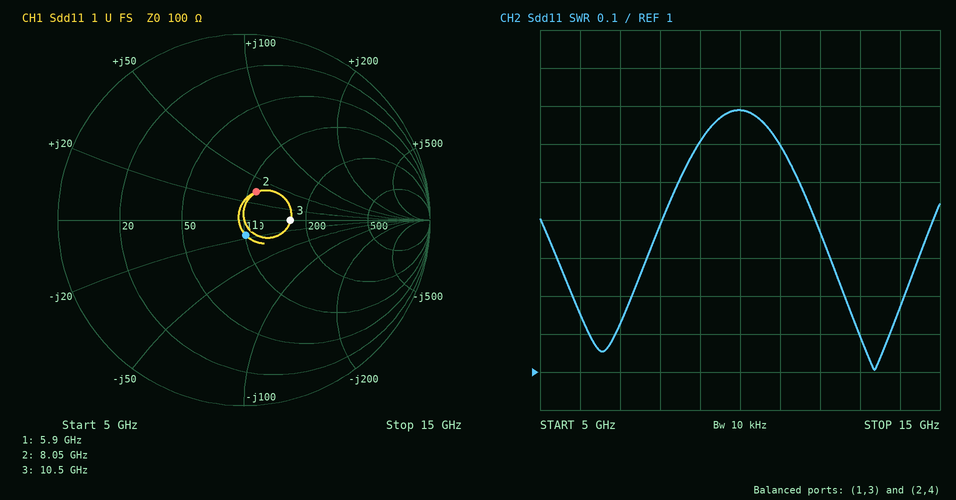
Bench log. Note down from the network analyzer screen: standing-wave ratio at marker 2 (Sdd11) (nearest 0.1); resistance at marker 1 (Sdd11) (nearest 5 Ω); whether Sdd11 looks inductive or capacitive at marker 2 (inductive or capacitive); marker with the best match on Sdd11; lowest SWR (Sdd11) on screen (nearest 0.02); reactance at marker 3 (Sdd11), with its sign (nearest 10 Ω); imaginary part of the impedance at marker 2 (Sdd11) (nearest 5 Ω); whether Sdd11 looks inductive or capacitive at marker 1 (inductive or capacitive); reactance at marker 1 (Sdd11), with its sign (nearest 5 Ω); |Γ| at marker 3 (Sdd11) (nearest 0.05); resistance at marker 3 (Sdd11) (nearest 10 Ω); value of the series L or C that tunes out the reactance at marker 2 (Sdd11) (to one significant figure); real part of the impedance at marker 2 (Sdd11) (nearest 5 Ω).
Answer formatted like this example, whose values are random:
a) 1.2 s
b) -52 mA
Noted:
a) 1.4
b) 100 Ω
c) inductive
d) marker 1
e) 1.00
f) 0 Ω
g) +35 Ω
h) capacitive
i) -15 Ω
j) 0.25
k) 170 Ω
l) 600 fF
m) 110 Ω
